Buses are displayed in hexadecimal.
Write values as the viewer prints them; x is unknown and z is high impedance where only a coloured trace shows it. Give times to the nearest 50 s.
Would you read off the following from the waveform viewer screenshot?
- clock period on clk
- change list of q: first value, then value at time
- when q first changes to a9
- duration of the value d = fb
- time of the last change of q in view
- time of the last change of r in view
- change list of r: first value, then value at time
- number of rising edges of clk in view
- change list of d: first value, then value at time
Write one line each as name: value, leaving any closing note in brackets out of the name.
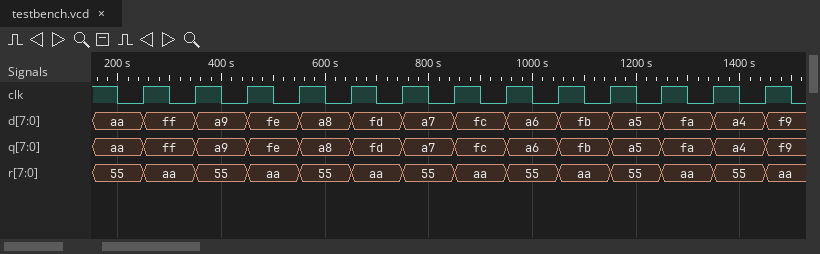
clock period on clk: 100 s
change list of q: first value, then value at time: aa, ff at 250 s, a9 at 350 s, fe at 450 s, a8 at 550 s, fd at 650 s, a7 at 750 s, fc at 850 s, a6 at 950 s, fb at 1050 s, a5 at 1150 s, fa at 1250 s, a4 at 1350 s, f9 at 1450 s
when q first changes to a9: 350 s
duration of the value d = fb: 100 s
time of the last change of q in view: 1450 s
time of the last change of r in view: 1450 s
change list of r: first value, then value at time: 55, aa at 250 s, 55 at 350 s, aa at 450 s, 55 at 550 s, aa at 650 s, 55 at 750 s, aa at 850 s, 55 at 950 s, aa at 1050 s, 55 at 1150 s, aa at 1250 s, 55 at 1350 s, aa at 1450 s
number of rising edges of clk in view: 13
change list of d: first value, then value at time: aa, ff at 250 s, a9 at 350 s, fe at 450 s, a8 at 550 s, fd at 650 s, a7 at 750 s, fc at 850 s, a6 at 950 s, fb at 1050 s, a5 at 1150 s, fa at 1250 s, a4 at 1350 s, f9 at 1450 s
